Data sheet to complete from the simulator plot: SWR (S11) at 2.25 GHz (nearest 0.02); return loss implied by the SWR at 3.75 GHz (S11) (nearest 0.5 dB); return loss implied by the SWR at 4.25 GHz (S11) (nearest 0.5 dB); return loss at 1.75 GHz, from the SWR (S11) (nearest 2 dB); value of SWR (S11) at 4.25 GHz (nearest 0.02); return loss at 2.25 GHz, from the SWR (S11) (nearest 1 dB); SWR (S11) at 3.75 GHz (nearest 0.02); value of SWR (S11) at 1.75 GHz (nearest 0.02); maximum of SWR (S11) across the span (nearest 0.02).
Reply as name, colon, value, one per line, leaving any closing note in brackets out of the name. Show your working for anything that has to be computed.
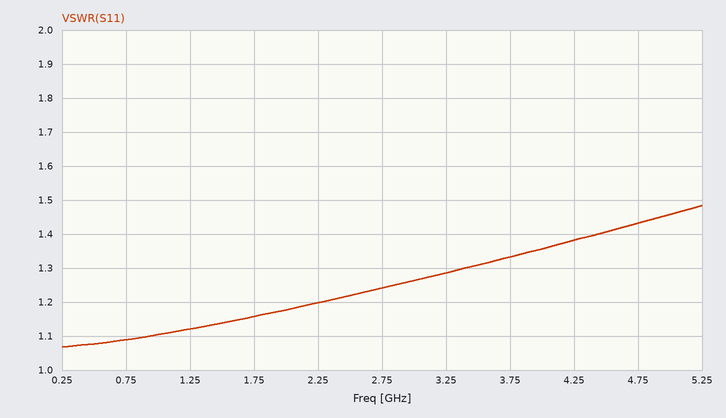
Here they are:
SWR (S11) at 2.25 GHz: 1.20
return loss implied by the SWR at 3.75 GHz (S11): −20 log10((1.34 − 1)/(1.34 + 1)) ≈ 16.8 dB, so 17.0 dB to the nearest 0.5 dB
return loss implied by the SWR at 4.25 GHz (S11): −20 log10((1.38 − 1)/(1.38 + 1)) ≈ 15.9 dB, so 16.0 dB to the nearest 0.5 dB
return loss at 1.75 GHz, from the SWR (S11): −20 log10((1.16 − 1)/(1.16 + 1)) ≈ 22.6 dB, so 22 dB to the nearest 2 dB
value of SWR (S11) at 4.25 GHz: 1.38
return loss at 2.25 GHz, from the SWR (S11): −20 log10((1.2 − 1)/(1.2 + 1)) ≈ 21 dB
SWR (S11) at 3.75 GHz: 1.34
value of SWR (S11) at 1.75 GHz: 1.16
maximum of SWR (S11) across the span: 1.48
